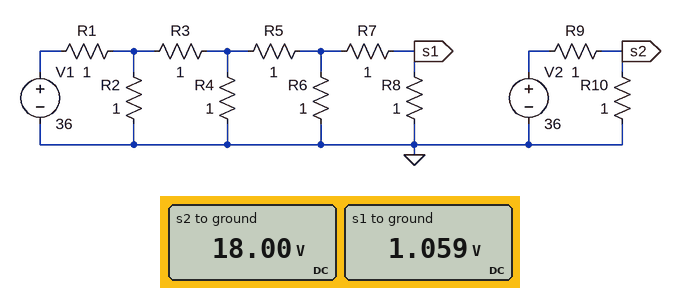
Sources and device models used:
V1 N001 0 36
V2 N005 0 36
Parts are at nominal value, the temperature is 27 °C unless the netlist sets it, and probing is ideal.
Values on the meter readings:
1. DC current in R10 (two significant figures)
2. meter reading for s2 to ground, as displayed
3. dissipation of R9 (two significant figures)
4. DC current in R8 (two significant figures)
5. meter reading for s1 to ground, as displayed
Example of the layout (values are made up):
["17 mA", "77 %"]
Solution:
["18 A", "18.00 V", "320 W", "1.1 A", "1.059 V"]
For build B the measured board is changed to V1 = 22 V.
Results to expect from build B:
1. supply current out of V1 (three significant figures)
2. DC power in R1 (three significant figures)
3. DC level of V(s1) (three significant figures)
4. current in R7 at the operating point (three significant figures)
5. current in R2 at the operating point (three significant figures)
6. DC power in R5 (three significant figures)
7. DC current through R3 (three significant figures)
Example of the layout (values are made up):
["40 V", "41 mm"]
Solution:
["13.6 A", "185 W", "647 mV", "647 mA", "8.41 A", "3.77 W", "5.18 A"]
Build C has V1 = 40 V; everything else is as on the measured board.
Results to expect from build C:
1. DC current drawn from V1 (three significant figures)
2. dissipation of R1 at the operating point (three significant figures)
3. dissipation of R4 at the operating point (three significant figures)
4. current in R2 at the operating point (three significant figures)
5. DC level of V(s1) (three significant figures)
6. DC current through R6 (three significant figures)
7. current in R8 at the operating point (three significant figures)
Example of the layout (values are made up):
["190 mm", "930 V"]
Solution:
["24.7 A", "610 W", "34.6 W", "15.3 A", "1.18 V", "2.35 A", "1.18 A"]
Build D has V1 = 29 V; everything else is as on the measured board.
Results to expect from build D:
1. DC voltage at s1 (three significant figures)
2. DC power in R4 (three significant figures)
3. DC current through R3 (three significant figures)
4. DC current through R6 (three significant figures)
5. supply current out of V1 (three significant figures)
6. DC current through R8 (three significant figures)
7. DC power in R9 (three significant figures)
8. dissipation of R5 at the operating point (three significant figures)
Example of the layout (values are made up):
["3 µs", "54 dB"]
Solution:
["853 mV", "18.2 W", "6.82 A", "1.71 A", "17.9 A", "853 mA", "324 W", "6.55 W"]
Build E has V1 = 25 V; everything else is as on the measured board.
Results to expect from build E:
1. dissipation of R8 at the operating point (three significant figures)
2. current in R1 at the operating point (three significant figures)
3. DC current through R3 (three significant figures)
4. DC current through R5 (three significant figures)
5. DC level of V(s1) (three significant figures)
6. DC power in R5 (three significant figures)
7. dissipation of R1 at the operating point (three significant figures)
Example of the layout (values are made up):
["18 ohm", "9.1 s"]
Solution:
["541 mW", "15.4 A", "5.88 A", "2.21 A", "735 mV", "4.87 W", "238 W"]
